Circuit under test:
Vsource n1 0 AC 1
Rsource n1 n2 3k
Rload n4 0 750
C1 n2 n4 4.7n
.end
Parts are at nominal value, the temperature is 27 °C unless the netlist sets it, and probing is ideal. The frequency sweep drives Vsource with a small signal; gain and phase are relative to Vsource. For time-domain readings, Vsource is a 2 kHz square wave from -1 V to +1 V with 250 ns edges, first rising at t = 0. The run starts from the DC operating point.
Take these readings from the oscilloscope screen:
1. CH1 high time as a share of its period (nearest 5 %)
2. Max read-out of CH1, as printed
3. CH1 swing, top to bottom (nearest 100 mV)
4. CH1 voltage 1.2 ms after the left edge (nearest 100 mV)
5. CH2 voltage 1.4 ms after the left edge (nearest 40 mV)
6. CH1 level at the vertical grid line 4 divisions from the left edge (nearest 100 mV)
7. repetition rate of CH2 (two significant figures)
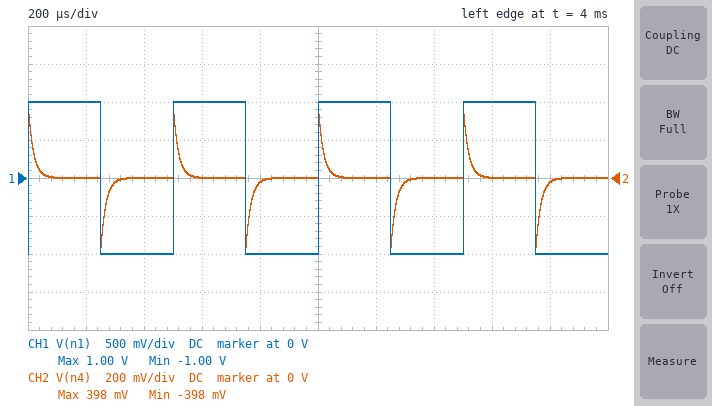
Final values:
50 %
1.00 V
2.0 V
1.0 V
0 V
-1.0 V
2.0 kHz
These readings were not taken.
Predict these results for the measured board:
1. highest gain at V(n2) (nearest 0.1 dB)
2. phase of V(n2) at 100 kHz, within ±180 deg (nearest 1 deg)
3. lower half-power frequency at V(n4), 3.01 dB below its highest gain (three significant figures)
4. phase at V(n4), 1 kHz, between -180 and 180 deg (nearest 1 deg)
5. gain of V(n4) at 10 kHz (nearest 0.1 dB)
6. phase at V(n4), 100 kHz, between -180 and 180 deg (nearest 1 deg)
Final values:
0 dB
-19 deg
9.03 kHz
84 deg
-16.6 dB
5 deg
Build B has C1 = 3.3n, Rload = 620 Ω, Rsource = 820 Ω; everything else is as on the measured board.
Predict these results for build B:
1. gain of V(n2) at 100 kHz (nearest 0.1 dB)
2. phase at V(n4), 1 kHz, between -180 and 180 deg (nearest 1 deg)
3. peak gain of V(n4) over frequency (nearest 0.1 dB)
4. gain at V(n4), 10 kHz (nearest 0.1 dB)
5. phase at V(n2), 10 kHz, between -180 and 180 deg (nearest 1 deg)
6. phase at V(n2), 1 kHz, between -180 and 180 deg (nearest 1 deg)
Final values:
-5.7 dB
88 deg
-7.3 dB
-18.2 dB
-9 deg
-1 deg
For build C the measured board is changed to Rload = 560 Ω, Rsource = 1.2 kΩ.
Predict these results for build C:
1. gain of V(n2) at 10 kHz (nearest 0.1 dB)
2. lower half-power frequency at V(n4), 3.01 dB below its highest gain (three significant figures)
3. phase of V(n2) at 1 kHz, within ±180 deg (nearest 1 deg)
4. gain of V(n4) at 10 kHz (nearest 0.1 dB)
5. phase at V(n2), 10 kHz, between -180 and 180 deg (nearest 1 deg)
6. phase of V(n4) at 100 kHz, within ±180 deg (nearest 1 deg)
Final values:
-0.9 dB
19.2 kHz
-2 deg
-16.7 dB
-18 deg
11 deg
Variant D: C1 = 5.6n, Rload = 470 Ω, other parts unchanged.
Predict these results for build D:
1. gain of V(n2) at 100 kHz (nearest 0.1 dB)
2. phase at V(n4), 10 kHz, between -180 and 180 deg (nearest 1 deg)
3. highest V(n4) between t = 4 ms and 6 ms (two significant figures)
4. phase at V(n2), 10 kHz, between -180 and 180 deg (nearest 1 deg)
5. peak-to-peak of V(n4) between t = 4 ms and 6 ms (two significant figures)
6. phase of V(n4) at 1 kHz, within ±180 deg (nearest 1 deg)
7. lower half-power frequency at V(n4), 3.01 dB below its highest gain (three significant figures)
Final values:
-16.0 dB
39 deg
270 mV
-41 deg
540 mV
83 deg
8.19 kHz
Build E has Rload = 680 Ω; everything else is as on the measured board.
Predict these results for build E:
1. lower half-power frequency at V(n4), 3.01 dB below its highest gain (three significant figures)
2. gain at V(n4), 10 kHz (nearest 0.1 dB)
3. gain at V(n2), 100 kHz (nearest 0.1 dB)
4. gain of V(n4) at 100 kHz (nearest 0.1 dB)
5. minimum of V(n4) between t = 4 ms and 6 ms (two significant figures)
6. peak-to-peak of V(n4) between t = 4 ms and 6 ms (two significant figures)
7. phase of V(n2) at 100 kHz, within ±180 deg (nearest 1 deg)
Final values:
9.20 kHz
-17.3 dB
-13.7 dB
-14.7 dB
-370 mV
730 mV
-21 deg
